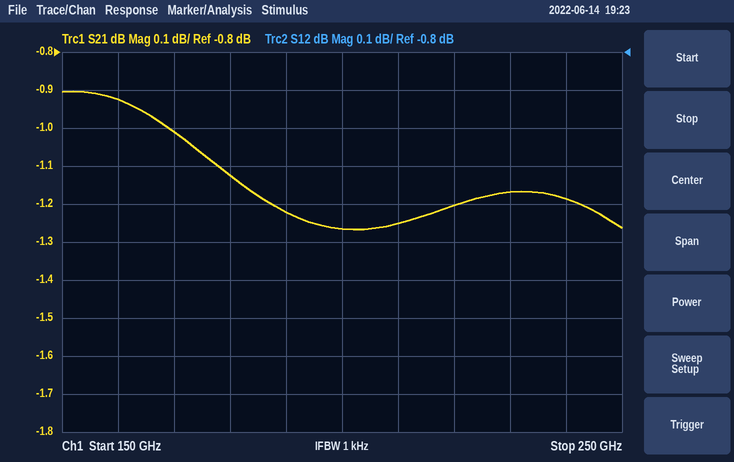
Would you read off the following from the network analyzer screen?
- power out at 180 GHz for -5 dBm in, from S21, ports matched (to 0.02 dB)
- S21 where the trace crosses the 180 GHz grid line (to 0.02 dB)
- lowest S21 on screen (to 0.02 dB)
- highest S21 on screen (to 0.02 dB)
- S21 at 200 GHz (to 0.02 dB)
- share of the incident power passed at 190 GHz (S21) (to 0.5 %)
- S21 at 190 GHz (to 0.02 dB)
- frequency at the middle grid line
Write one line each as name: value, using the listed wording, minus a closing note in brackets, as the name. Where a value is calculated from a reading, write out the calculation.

power out at 180 GHz for -5 dBm in, from S21, ports matched: -5 dBm + (-1.12 dB) = -6.12 dBm
S21 where the trace crosses the 180 GHz grid line: -1.12 dB
lowest S21 on screen: -1.26 dB
highest S21 on screen: -0.90 dB
S21 at 200 GHz: -1.26 dB
share of the incident power passed at 190 GHz (S21): 10^(-1.22/10) ≈ 75.5 %
S21 at 190 GHz: -1.22 dB
frequency at the middle grid line: 200 GHz
